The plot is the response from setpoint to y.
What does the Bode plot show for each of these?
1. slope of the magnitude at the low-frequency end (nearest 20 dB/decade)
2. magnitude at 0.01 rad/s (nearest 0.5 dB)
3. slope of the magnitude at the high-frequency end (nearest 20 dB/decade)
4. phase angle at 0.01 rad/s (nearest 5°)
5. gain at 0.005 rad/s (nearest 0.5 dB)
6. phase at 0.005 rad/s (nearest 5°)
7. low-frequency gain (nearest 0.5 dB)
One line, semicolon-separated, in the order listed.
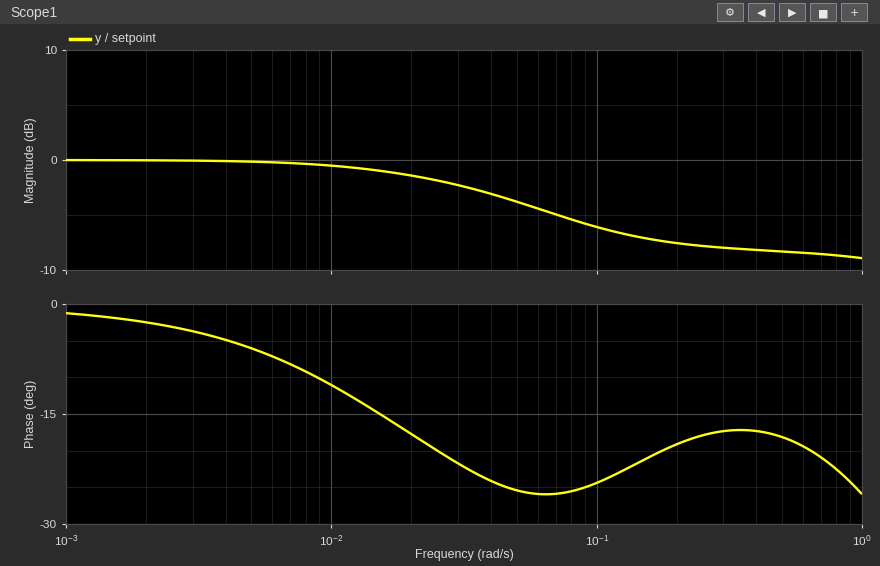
0 dB/decade; -0.5 dB; 0 dB/decade; -10°; 0.0 dB; -5°; 0.0 dB
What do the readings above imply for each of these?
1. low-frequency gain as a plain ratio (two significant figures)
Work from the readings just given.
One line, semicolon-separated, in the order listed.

1.0
